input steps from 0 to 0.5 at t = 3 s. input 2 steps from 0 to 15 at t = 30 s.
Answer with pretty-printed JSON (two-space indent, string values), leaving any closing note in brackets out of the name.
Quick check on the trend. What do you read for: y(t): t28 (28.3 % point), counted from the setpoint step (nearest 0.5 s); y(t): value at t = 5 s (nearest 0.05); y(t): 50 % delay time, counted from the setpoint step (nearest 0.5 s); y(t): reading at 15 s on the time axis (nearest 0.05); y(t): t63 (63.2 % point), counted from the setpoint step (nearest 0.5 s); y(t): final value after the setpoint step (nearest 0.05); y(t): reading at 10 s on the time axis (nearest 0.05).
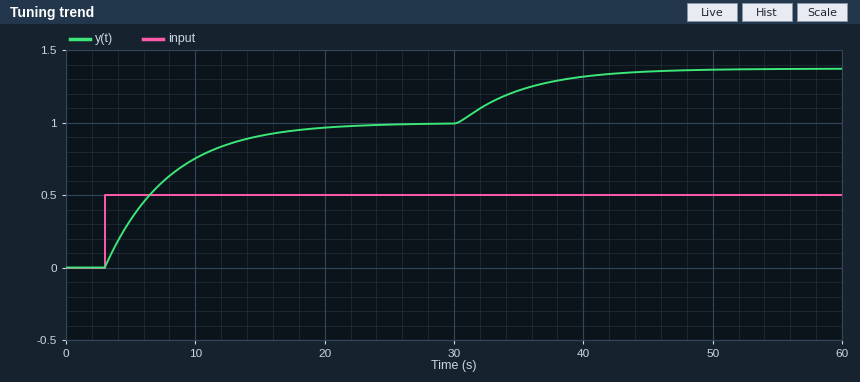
{
  "y(t): t28 (28.3 % point), counted from the setpoint step": "1.5 s",
  "y(t): value at t = 5 s": "0.35",
  "y(t): 50 % delay time, counted from the setpoint step": "3.5 s",
  "y(t): reading at 15 s on the time axis": "0.90",
  "y(t): t63 (63.2 % point), counted from the setpoint step": "5.0 s",
  "y(t): final value after the setpoint step": "1.00",
  "y(t): reading at 10 s on the time axis": "0.75"
}
